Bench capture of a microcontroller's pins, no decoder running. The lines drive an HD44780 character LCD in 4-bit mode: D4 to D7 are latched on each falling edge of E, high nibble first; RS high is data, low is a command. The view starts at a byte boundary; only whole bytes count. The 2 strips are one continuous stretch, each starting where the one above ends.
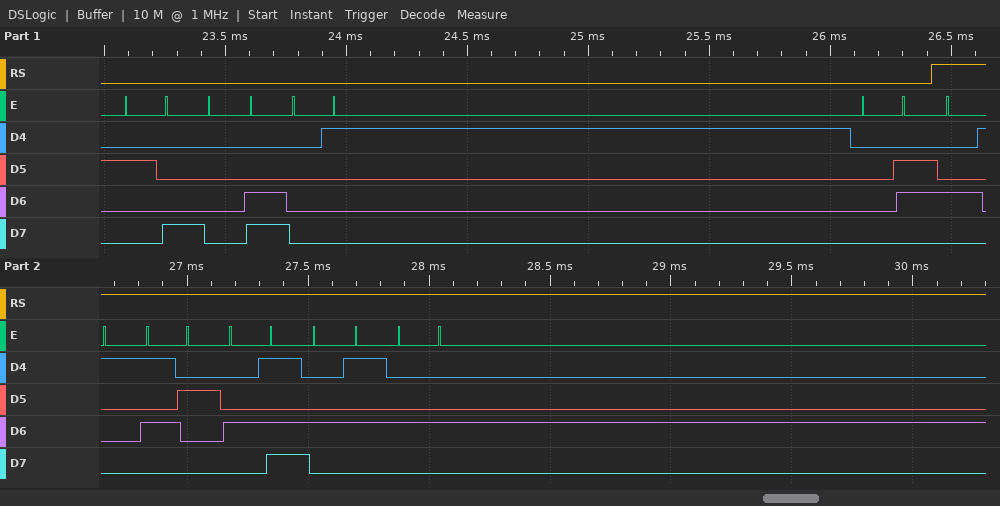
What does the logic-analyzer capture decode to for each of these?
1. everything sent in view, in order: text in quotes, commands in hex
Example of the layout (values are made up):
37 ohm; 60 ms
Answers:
0x28 0x0C 0x01 0x06 "ARMED"
